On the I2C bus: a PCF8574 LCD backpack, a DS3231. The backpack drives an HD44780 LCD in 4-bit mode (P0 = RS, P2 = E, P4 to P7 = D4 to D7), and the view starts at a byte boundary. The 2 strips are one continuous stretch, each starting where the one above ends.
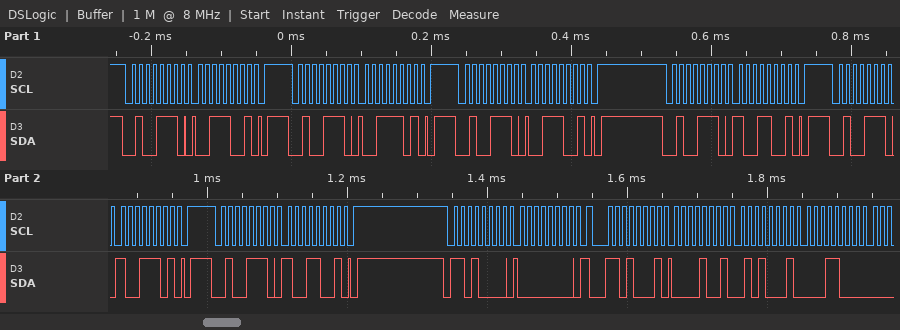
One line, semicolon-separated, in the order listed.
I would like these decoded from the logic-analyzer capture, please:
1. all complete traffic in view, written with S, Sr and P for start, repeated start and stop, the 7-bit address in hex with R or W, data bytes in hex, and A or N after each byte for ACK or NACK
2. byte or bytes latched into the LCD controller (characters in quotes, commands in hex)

S 27W A 39 A P S 27W A 3D A P S 27W A 39 A P S 27W A 99 A P S 27W A 9D A P S 27W A 99 A P S 68W A 00 A Sr 68R A 09 A 51 A 18 A; '9'
